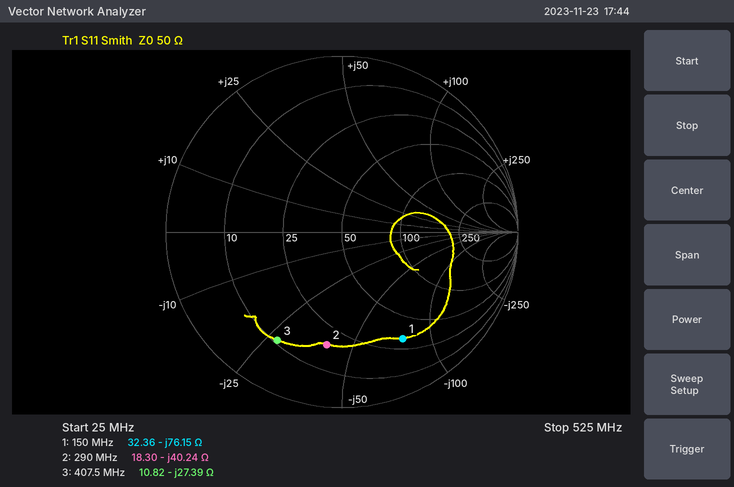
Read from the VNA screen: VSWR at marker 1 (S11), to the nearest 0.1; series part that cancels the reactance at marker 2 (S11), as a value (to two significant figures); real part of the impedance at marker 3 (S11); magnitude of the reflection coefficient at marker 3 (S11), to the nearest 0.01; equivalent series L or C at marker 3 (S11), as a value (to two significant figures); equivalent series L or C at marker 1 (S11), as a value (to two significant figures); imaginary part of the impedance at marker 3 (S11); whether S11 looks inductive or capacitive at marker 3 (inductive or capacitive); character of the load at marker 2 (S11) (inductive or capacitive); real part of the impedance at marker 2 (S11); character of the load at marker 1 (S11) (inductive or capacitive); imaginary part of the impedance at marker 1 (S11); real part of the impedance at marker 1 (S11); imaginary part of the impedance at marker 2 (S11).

5.6
22 nH
10.82 Ω
0.72
14 pF
14 pF
-27.39 Ω
capacitive
capacitive
18.30 Ω
capacitive
-76.15 Ω
32.36 Ω
-40.24 Ω
